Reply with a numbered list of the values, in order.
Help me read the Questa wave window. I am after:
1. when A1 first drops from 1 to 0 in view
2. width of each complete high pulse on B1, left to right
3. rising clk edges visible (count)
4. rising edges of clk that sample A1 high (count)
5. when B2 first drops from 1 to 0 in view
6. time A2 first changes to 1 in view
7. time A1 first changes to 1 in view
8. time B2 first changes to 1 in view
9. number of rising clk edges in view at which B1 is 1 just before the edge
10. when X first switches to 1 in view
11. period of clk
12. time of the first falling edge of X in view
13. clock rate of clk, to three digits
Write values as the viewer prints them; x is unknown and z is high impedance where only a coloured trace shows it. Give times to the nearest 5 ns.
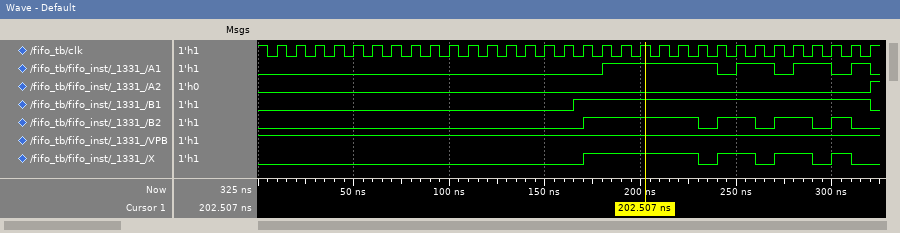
1. 240 ns
2. 155 ns
3. 32
4. 11
5. 230 ns
6. 320 ns
7. 180 ns
8. 170 ns
9. 16
10. 170 ns
11. 10 ns
12. 230 ns
13. 100 MHz
